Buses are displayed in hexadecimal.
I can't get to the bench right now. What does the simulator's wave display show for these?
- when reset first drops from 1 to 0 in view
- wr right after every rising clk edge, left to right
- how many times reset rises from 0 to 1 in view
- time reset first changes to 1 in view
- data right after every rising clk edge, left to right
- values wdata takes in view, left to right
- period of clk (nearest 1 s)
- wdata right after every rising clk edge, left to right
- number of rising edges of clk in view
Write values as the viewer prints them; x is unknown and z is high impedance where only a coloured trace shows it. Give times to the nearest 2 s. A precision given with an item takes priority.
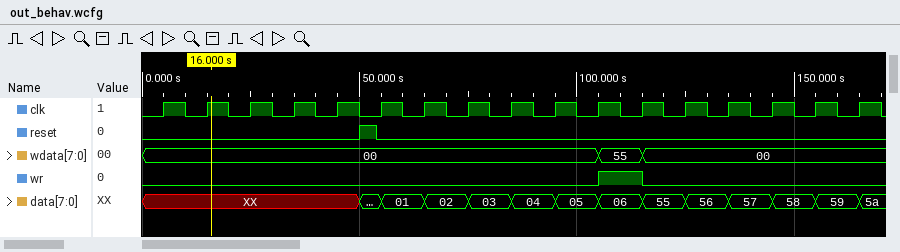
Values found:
54 s
0 0 0 0 0 0 0 0 0 0 1 0 0 0 0 0 0
1
50 s
XX, XX, XX, XX, XX, 01, 02, 03, 04, 05, 06, 55, 56, 57, 58, 59, 5a
00, 55, 00
10 s
00, 00, 00, 00, 00, 00, 00, 00, 00, 00, 55, 00, 00, 00, 00, 00, 00
17
